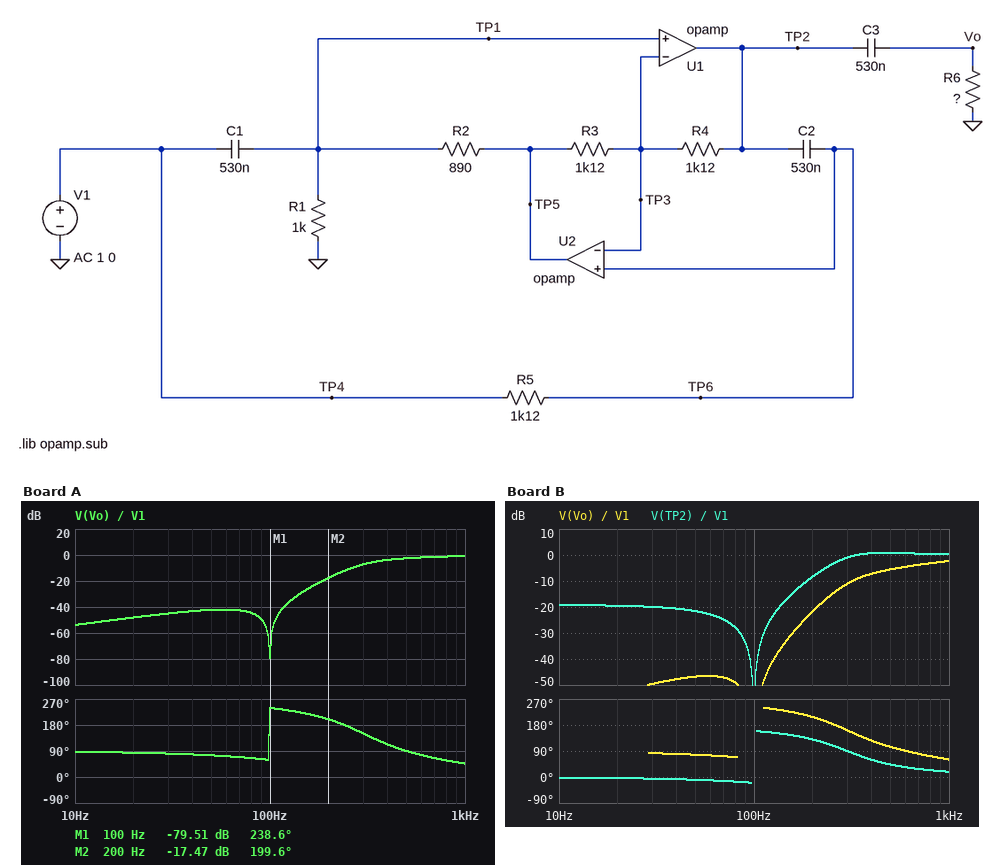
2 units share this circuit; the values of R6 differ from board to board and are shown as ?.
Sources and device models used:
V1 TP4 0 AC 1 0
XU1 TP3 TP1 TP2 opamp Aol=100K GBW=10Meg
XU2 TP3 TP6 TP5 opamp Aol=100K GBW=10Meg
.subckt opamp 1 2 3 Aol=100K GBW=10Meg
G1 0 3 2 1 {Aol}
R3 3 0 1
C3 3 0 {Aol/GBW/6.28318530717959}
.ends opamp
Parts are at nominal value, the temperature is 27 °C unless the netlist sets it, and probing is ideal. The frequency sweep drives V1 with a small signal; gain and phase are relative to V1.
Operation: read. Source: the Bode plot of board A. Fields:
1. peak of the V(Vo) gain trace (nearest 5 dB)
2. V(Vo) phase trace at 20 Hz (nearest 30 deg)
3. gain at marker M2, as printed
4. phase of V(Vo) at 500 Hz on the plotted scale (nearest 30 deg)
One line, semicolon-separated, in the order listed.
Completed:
0 dB; 90 deg; -17.47 dB; 90 deg
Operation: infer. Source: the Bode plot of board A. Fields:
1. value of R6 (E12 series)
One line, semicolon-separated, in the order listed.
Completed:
560 Ω
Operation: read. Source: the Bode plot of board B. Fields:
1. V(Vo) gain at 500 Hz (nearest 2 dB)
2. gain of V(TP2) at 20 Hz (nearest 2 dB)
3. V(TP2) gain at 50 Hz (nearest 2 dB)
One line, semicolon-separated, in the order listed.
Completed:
-6 dB; -20 dB; -22 dB
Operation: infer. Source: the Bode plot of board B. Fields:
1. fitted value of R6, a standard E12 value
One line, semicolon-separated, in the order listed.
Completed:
330 Ω
